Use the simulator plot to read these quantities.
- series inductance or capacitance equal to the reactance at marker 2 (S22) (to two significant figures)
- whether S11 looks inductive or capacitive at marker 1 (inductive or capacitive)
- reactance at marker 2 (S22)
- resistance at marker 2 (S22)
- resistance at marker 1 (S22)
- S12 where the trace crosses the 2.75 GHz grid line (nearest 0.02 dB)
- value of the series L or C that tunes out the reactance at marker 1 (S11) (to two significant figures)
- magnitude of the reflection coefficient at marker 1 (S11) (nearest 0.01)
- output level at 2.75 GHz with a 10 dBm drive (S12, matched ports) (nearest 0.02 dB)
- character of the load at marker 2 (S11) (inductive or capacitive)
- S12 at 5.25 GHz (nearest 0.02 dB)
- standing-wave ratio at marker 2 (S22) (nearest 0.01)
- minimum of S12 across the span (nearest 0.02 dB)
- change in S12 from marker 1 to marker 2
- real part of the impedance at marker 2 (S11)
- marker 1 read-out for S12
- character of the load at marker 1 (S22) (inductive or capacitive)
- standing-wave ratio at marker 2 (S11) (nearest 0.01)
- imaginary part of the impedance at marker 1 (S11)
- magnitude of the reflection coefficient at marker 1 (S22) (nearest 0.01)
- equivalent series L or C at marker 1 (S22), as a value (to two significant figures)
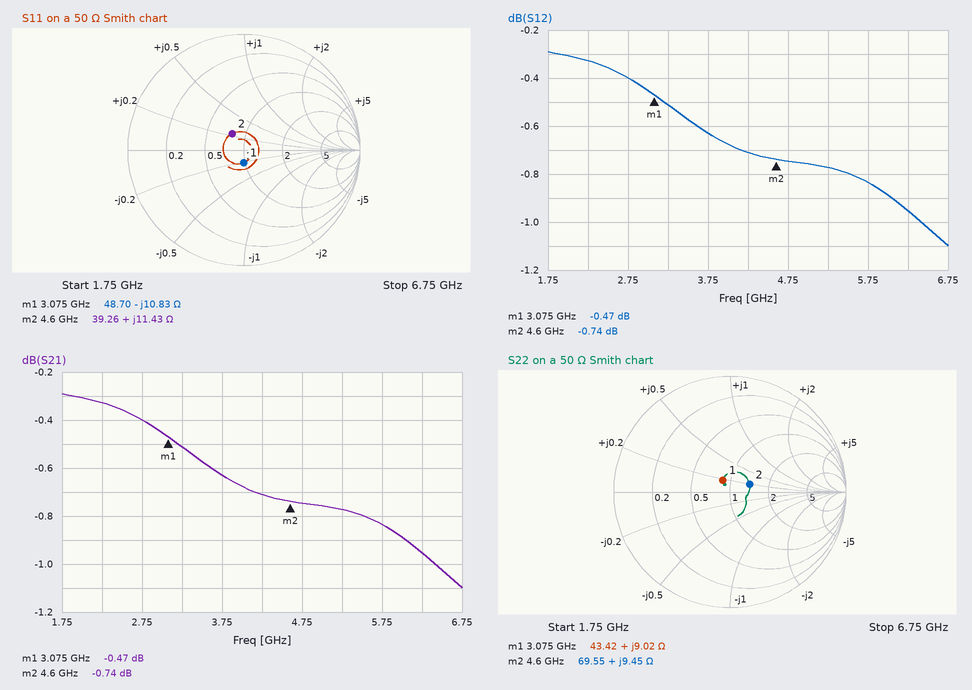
330 pH
capacitive
+9.45 Ω
69.55 Ω
43.42 Ω
-0.40 dB
560 pH
0.11
9.60 dBm
inductive
-0.78 dB
1.44
-1.10 dB
-0.27 dB
39.26 Ω
-0.47 dB
inductive
1.42
-10.83 Ω
0.12
470 pH
